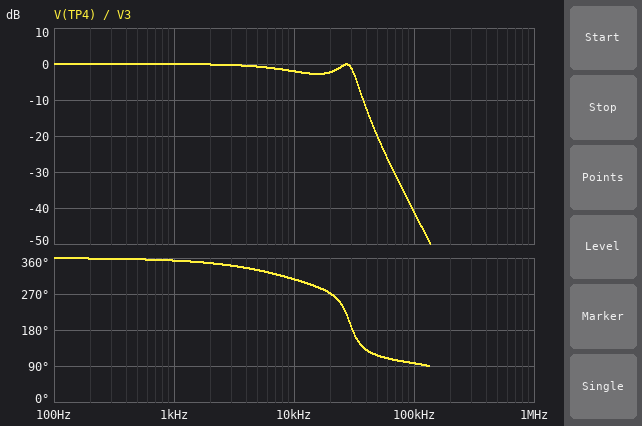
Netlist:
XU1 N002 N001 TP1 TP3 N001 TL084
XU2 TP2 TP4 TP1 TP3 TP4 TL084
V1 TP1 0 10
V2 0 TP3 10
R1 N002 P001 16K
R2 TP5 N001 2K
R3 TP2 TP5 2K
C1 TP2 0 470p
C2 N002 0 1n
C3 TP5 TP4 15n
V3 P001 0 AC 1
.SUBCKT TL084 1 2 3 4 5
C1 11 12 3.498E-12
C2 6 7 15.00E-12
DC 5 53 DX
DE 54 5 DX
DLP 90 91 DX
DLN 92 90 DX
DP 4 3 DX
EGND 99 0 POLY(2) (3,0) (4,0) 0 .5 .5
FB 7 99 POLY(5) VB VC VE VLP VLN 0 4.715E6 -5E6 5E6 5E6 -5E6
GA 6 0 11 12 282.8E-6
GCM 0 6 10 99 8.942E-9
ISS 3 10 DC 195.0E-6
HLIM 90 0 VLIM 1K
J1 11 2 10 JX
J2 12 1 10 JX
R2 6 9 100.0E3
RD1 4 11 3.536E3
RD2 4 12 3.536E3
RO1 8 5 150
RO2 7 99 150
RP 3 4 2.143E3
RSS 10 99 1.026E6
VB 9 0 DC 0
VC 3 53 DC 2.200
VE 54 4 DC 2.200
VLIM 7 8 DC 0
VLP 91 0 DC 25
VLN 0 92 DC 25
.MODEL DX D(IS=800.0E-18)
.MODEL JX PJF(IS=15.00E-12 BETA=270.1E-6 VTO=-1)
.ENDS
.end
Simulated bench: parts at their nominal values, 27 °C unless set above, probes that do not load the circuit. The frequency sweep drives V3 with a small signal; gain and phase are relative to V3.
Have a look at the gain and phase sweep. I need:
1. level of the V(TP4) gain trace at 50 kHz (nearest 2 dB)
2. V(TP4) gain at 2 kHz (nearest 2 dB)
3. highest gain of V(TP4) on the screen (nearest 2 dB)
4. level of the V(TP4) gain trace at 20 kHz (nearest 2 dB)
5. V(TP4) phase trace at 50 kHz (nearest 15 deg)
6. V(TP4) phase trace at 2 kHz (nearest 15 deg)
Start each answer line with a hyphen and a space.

- -20 dB
- 0 dB
- 0 dB
- -2 dB
- 120 deg
- 345 deg
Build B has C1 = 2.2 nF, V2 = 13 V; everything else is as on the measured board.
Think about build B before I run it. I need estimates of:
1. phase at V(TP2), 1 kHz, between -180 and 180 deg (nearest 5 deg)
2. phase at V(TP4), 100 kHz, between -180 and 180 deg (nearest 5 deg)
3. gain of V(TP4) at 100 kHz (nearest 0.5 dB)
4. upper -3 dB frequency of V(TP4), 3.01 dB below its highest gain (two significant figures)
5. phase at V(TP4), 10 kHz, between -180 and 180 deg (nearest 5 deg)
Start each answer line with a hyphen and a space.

- -10 deg
- 90 deg
- -54.5 dB
- 14 kHz
- -95 deg
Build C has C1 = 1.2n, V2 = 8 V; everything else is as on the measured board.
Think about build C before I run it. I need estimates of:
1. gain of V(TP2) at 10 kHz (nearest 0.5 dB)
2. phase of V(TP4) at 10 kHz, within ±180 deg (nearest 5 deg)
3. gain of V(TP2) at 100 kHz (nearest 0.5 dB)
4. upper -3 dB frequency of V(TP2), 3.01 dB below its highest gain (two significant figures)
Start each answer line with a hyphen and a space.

- -1.0 dB
- -70 deg
- -49.5 dB
- 20 kHz
